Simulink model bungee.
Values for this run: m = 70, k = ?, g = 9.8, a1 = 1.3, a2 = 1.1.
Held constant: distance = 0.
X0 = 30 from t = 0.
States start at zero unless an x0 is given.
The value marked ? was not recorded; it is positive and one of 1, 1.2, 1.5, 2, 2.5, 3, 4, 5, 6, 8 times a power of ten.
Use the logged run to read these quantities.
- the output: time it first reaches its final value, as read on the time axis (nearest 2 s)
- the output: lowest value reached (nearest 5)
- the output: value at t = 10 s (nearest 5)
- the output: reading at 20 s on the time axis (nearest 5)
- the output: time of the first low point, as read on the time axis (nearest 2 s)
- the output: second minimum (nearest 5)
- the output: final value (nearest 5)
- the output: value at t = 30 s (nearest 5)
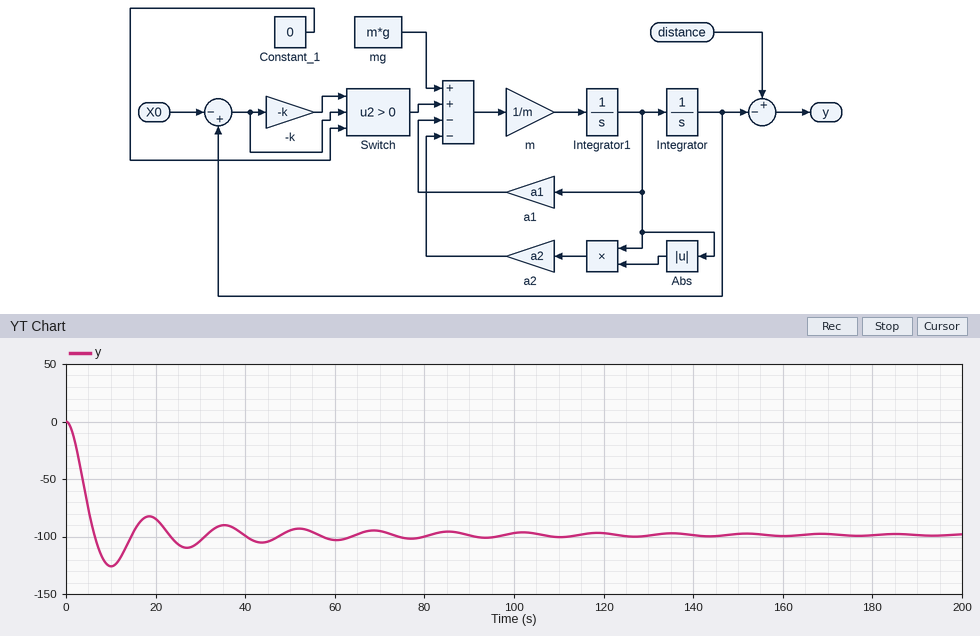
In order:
6 s
-125
-125
-85
10 s
-110
-100
-105
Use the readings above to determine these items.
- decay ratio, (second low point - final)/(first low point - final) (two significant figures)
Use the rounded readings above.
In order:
0.40
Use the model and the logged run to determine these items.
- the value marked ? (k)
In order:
10
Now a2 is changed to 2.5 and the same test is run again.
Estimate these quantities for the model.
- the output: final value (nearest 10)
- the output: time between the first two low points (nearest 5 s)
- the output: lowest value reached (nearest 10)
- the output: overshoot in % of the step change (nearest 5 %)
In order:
-100
15 s
-110
15 %
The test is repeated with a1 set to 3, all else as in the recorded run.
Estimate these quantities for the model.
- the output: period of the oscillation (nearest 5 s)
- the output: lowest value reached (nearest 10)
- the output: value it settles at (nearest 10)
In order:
15 s
-120
-100
